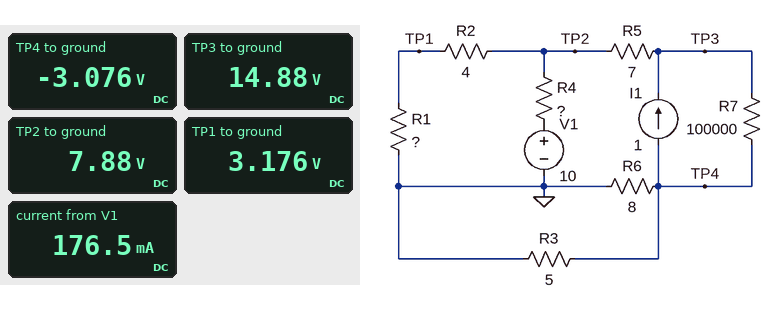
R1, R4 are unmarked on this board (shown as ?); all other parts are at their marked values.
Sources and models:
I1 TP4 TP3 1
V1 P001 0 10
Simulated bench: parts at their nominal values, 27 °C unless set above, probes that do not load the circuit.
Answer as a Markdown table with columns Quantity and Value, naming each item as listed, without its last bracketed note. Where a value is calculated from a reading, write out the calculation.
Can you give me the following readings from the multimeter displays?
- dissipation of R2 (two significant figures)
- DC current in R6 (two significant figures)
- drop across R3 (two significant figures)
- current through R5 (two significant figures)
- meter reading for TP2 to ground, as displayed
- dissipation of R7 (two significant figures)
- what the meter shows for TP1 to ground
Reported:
| Quantity | Value |
|---|---|
| dissipation of R2 | (7.88 V - 3.176 V)^2 / 4 Ω = 5.5 W |
| DC current in R6 | (0 V - (-3.076 V)) / 8 Ω = 380 mA |
| drop across R3 | 0 V - (-3.076 V) = 3.1 V |
| current through R5 | (14.88 V - 7.88 V) / 7 Ω = 1.0 A |
| meter reading for TP2 to ground, as displayed | 7.88 V |
| dissipation of R7 | (14.88 V - (-3.076 V))^2 / 100 kΩ = 3.2 mW |
| what the meter shows for TP1 to ground | 3.176 V |
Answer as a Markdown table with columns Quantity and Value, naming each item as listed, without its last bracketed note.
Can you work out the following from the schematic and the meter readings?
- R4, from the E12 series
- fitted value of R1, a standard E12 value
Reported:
| Quantity | Value |
|---|---|
| R4, from the E12 series | 12 Ω |
| fitted value of R1, a standard E12 value | 2.7 Ω |
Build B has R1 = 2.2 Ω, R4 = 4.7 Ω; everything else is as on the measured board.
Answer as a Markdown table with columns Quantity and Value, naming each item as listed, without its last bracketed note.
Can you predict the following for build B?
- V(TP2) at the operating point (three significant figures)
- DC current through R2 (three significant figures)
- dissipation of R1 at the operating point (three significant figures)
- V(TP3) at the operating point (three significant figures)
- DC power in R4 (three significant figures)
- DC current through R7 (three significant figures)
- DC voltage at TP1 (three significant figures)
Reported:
| Quantity | Value |
|---|---|
| V(TP2) at the operating point | 8.36 V |
| DC current through R2 | 1.35 A |
| dissipation of R1 at the operating point | 4.00 W |
| V(TP3) at the operating point | 15.4 V |
| DC power in R4 | 572 mW |
| DC current through R7 | 184 µA |
| DC voltage at TP1 | 2.97 V |
